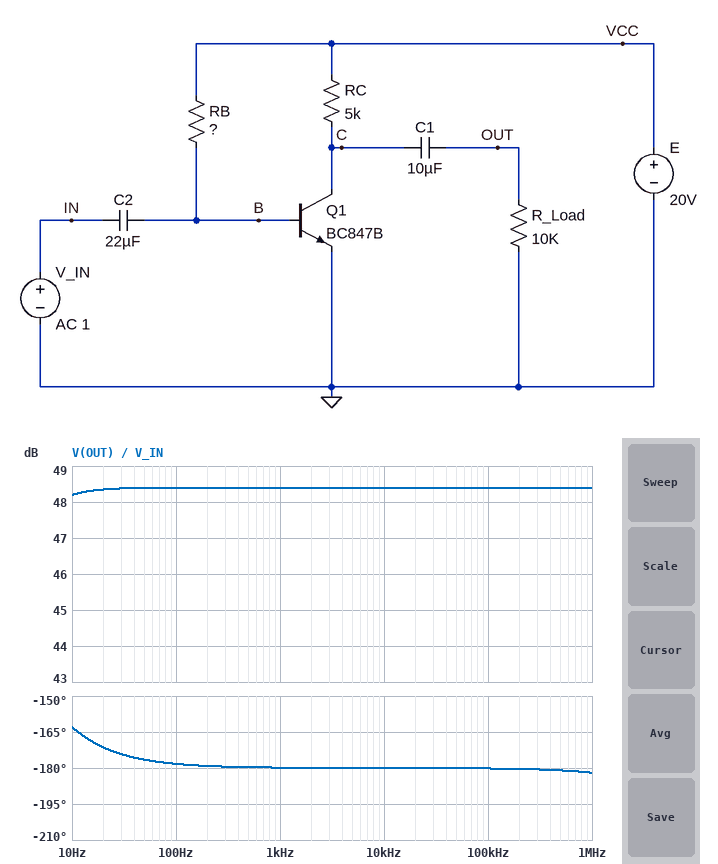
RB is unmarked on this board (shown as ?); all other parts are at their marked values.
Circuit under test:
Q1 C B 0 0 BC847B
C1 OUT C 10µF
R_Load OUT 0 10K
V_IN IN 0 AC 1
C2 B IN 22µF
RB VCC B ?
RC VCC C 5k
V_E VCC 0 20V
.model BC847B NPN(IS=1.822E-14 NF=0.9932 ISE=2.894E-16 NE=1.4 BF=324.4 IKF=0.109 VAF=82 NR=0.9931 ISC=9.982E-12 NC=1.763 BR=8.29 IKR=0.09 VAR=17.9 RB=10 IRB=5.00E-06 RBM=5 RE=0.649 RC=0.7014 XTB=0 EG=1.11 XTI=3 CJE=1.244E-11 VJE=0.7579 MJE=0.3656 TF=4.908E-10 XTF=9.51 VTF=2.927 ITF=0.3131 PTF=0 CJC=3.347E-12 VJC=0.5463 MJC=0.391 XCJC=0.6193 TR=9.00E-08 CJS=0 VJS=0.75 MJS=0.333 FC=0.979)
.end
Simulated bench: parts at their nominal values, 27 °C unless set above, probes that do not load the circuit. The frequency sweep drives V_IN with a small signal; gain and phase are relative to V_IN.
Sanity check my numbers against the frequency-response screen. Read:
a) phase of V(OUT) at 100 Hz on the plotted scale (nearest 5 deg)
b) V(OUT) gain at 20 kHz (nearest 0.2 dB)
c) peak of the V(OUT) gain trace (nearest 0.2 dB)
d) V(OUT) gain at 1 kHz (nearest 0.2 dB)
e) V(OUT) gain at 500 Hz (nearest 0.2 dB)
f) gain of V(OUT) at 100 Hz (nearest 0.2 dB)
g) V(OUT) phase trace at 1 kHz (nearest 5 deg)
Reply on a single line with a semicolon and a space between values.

-180 deg; 48.4 dB; 48.4 dB; 48.4 dB; 48.4 dB; 48.4 dB; -180 deg
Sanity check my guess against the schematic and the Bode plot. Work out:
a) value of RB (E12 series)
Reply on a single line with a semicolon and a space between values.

2.7 MΩ
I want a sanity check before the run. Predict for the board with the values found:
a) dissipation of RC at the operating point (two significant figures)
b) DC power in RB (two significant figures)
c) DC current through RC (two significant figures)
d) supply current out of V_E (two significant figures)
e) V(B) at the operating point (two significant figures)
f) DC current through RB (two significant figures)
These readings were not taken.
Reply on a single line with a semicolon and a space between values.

29 mW; 140 µW; 2.4 mA; 2.4 mA; 660 mV; 7.2 µA
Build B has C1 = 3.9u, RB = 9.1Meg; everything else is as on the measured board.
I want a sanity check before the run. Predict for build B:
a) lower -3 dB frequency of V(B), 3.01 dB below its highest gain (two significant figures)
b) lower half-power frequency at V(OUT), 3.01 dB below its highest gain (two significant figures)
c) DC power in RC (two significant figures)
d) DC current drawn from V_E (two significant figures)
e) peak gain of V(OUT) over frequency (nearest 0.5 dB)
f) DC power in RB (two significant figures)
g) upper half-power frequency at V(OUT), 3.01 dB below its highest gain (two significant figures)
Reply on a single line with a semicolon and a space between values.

590 mHz; 2.9 Hz; 3.1 mW; 790 µA; 39.5 dB; 41 µW; 47 MHz
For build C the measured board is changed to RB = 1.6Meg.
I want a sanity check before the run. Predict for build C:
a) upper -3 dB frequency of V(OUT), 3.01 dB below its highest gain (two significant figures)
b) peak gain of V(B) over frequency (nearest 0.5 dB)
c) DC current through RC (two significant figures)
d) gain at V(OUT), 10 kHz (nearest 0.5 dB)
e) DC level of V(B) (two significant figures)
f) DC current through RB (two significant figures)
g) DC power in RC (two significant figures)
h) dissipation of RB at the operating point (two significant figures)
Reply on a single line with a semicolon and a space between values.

15 MHz; 0 dB; 3.7 mA; 51.5 dB; 670 mV; 12 µA; 68 mW; 230 µW
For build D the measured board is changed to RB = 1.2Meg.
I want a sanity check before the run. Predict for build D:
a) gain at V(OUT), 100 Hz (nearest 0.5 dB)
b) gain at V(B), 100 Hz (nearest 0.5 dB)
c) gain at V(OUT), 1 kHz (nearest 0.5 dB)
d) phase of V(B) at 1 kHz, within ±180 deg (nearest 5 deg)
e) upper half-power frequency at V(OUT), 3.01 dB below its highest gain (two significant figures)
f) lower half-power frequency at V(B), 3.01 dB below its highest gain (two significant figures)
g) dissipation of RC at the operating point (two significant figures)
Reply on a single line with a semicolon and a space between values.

40.0 dB; -2.5 dB; 42.5 dB; 5 deg; 1.4 MHz; 91 Hz; 79 mW
